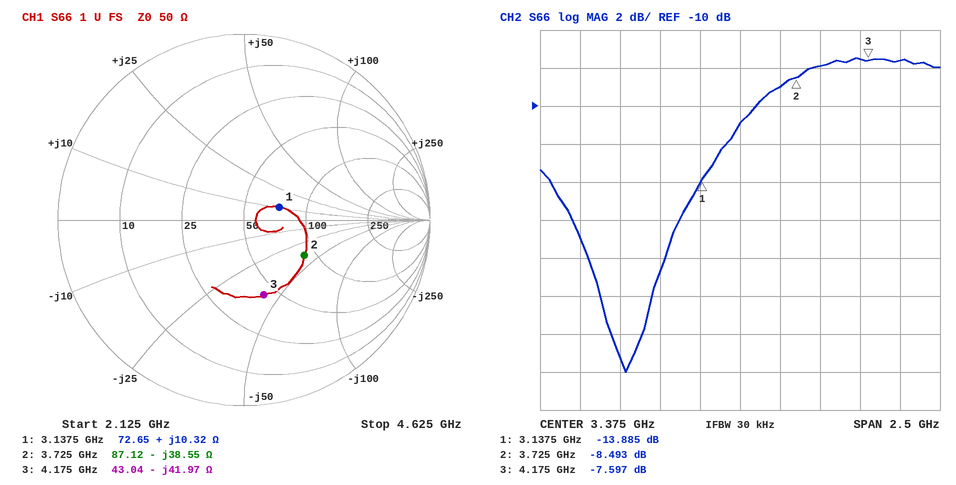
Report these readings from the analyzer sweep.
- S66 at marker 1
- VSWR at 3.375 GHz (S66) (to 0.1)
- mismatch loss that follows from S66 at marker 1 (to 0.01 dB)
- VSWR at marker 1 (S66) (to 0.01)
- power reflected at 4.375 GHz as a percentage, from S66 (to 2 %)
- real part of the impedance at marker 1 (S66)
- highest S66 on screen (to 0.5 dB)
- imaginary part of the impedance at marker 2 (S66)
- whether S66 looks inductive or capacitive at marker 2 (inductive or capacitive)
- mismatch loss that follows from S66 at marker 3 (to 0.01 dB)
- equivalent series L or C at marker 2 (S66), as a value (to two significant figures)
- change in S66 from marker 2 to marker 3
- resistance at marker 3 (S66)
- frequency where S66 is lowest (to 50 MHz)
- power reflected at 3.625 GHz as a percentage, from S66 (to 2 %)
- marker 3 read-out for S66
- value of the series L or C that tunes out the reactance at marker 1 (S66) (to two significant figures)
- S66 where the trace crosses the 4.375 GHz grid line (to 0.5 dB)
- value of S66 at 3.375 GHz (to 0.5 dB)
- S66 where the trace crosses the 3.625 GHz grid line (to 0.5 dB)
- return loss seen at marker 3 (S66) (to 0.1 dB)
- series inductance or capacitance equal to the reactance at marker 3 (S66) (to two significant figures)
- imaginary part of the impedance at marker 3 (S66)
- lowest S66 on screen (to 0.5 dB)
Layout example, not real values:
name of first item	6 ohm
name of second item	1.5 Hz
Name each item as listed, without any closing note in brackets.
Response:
S66 at marker 1	-13.885 dB
VSWR at 3.375 GHz (S66)	1.8
mismatch loss that follows from S66 at marker 1	0.18 dB
VSWR at marker 1 (S66)	1.51
power reflected at 4.375 GHz as a percentage, from S66	18 %
real part of the impedance at marker 1	72.65 Ω
highest S66 on screen	-7.5 dB
imaginary part of the impedance at marker 2	-38.55 Ω
whether S66 looks inductive or capacitive at marker 2	capacitive
mismatch loss that follows from S66 at marker 3	0.83 dB
equivalent series L or C at marker 2 (S66), as a value	1.1 pF
change in S66 from marker 2 to marker 3	0.896 dB
resistance at marker 3	43.04 Ω
frequency where S66 is lowest	2.65 GHz
power reflected at 3.625 GHz as a percentage, from S66	12 %
marker 3 read-out for S66	-7.597 dB
value of the series L or C that tunes out the reactance at marker 1 (S66)	4.9 pF
S66 where the trace crosses the 4.375 GHz grid line	-7.5 dB
value of S66 at 3.375 GHz	-11.0 dB
S66 where the trace crosses the 3.625 GHz grid line	-9.0 dB
return loss seen at marker 3 (S66)	7.6 dB
series inductance or capacitance equal to the reactance at marker 3 (S66)	910 fF
imaginary part of the impedance at marker 3	-41.97 Ω
lowest S66 on screen	-24.0 dB
